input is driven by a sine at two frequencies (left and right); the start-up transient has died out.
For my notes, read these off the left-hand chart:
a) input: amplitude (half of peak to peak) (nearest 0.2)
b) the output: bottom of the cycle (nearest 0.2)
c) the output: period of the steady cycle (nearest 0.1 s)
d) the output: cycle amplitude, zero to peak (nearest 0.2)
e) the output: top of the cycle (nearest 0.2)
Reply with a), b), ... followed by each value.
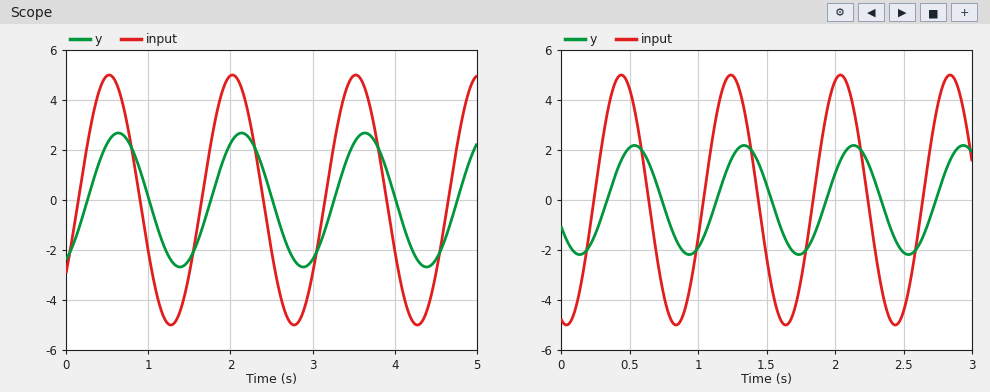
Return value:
a) 5.0
b) -2.6
c) 1.5 s
d) 2.6
e) 2.6
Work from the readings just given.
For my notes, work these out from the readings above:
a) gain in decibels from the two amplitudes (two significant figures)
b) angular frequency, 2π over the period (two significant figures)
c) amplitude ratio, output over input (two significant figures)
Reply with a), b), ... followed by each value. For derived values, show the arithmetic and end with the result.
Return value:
a) 20 log10(2.6 / 5) = -5.7 dB
b) 2π / 1.5 = 4.2 rad/s
c) 2.6 / 5 = 0.52
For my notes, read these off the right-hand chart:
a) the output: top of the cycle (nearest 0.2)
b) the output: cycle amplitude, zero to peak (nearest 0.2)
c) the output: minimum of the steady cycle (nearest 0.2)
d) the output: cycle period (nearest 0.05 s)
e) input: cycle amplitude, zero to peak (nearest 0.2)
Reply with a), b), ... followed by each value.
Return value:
a) 2.2
b) 2.2
c) -2.2
d) 0.80 s
e) 5.0
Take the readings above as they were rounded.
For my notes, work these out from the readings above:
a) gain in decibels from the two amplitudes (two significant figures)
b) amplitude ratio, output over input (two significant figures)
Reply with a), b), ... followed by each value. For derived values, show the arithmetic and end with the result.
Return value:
a) 20 log10(2.2 / 5) = -7.1 dB
b) 2.2 / 5 = 0.44
